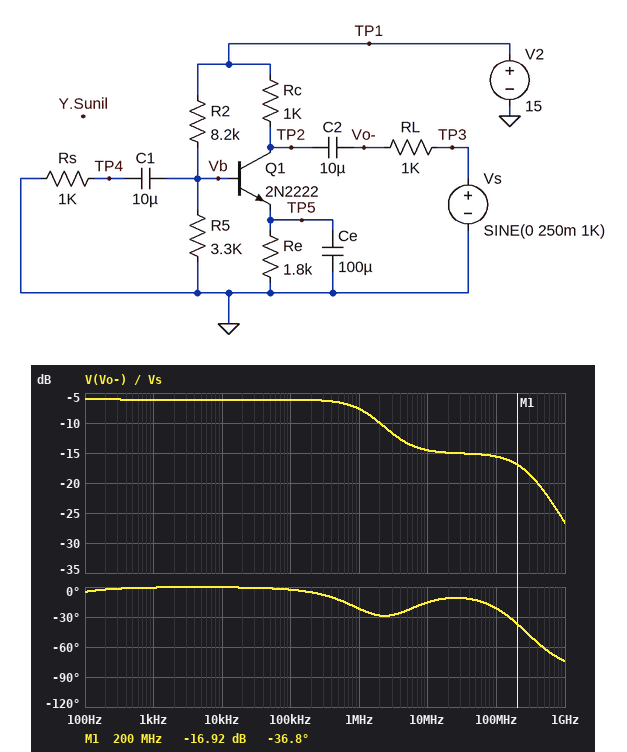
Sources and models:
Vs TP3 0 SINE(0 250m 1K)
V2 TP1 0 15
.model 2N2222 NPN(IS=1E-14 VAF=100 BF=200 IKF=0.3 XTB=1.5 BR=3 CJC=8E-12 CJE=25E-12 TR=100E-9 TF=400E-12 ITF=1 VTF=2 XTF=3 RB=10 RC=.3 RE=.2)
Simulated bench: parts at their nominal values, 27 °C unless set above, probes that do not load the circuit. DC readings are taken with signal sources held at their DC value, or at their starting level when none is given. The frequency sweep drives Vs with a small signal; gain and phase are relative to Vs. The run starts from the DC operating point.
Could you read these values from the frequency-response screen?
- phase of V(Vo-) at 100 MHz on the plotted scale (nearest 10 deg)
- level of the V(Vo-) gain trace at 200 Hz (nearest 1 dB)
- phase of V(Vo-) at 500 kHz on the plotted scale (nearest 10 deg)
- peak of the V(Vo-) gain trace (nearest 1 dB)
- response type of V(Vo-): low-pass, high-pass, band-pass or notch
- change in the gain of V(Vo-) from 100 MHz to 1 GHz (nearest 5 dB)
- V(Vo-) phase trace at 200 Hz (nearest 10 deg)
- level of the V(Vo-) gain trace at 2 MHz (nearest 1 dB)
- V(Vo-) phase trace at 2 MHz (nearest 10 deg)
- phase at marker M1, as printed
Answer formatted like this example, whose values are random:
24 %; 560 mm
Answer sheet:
-20 deg; -6 dB; -10 deg; -6 dB; low-pass; -10 dB; 0 deg; -10 dB; -30 deg; -36.8 deg
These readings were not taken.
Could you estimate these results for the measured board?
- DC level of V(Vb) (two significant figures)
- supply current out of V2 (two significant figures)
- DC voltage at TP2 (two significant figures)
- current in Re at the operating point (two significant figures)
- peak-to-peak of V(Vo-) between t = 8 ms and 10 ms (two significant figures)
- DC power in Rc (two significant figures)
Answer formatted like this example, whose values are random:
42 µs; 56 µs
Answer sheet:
4.3 V; 3.3 mA; 13 V; 2.0 mA; 250 mV; 4.0 mW
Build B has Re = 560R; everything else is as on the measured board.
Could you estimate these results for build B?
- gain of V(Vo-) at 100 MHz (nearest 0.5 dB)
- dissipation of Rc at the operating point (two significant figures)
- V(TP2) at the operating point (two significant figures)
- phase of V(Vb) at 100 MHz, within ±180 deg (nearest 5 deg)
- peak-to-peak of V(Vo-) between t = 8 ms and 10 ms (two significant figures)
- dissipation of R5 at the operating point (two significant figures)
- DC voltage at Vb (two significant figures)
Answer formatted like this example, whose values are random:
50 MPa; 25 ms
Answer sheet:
-19.5 dB; 39 mW; 8.7 V; -15 deg; 240 mV; 5.4 mW; 4.2 V
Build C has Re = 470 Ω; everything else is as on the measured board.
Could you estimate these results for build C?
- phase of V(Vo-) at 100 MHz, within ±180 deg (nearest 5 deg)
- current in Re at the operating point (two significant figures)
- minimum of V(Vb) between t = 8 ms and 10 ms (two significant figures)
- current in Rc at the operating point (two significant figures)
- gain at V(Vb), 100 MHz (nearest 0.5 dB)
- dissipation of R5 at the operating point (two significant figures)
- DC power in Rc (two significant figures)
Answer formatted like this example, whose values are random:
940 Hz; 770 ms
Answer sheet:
-15 deg; 7.5 mA; 4.2 V; 7.4 mA; -51.0 dB; 5.4 mW; 55 mW
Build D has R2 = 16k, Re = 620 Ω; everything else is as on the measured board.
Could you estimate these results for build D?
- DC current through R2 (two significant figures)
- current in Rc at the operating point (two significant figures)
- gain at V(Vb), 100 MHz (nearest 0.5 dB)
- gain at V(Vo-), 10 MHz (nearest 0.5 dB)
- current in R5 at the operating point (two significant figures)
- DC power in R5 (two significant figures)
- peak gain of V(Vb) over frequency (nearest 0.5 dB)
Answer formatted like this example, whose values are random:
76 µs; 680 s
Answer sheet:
780 µA; 3.0 mA; -45.0 dB; -15.5 dB; 770 µA; 1.9 mW; -44.5 dB
